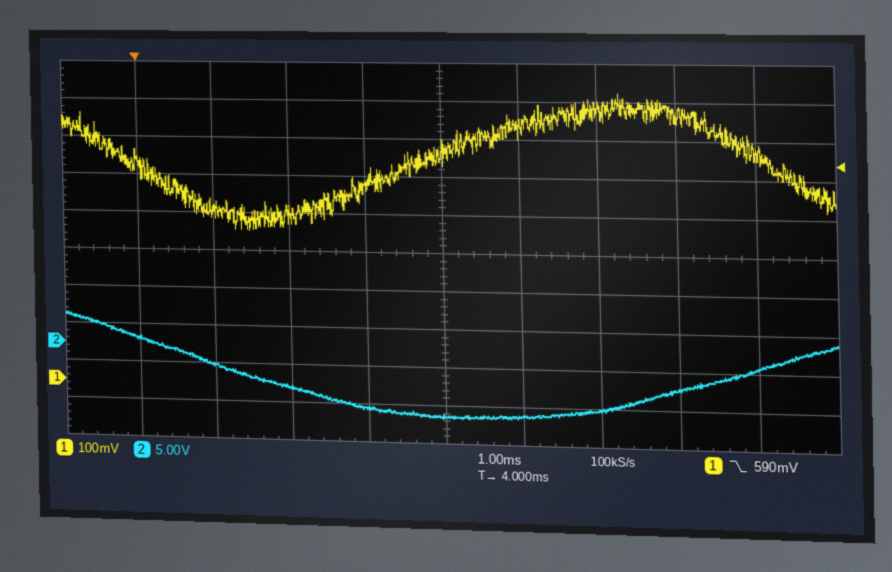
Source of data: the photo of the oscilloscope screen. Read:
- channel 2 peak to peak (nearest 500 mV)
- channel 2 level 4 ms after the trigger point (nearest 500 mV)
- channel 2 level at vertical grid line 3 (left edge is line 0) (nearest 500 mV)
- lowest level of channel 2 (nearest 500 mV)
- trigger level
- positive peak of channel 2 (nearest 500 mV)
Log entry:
13.0 V
-9.0 V
-5.5 V
-9.0 V
590 mV
4.0 V
